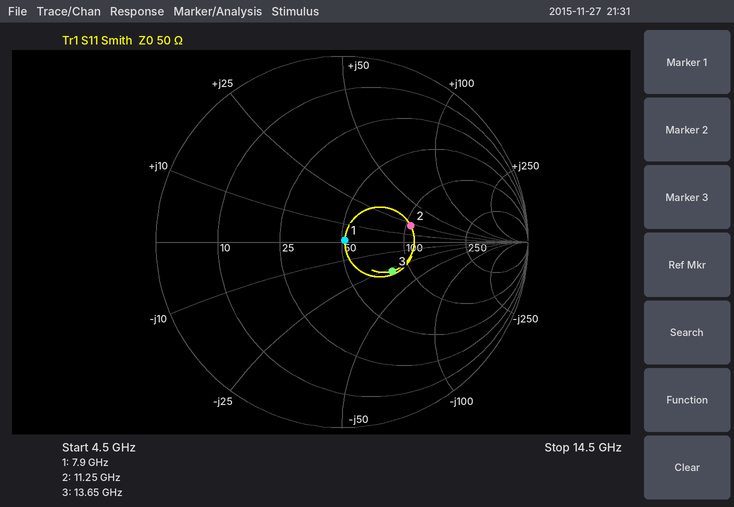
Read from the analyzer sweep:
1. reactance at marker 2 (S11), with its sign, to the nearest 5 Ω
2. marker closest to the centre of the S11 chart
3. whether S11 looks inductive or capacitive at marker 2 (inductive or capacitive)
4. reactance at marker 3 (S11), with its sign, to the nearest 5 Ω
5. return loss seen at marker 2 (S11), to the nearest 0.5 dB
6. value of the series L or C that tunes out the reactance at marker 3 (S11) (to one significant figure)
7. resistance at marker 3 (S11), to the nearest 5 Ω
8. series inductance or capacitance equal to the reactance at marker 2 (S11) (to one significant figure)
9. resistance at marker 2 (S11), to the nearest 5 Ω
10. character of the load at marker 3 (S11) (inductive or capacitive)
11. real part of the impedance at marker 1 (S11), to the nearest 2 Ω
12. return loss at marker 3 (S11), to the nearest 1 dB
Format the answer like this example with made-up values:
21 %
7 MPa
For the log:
+20 Ω
marker 1
inductive
-30 Ω
8.5 dB
300 pH
80 Ω
300 pH
105 Ω
capacitive
52 Ω
10 dB
